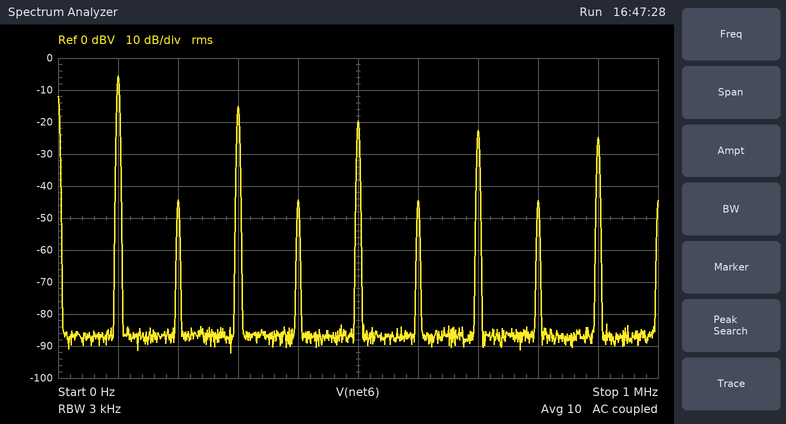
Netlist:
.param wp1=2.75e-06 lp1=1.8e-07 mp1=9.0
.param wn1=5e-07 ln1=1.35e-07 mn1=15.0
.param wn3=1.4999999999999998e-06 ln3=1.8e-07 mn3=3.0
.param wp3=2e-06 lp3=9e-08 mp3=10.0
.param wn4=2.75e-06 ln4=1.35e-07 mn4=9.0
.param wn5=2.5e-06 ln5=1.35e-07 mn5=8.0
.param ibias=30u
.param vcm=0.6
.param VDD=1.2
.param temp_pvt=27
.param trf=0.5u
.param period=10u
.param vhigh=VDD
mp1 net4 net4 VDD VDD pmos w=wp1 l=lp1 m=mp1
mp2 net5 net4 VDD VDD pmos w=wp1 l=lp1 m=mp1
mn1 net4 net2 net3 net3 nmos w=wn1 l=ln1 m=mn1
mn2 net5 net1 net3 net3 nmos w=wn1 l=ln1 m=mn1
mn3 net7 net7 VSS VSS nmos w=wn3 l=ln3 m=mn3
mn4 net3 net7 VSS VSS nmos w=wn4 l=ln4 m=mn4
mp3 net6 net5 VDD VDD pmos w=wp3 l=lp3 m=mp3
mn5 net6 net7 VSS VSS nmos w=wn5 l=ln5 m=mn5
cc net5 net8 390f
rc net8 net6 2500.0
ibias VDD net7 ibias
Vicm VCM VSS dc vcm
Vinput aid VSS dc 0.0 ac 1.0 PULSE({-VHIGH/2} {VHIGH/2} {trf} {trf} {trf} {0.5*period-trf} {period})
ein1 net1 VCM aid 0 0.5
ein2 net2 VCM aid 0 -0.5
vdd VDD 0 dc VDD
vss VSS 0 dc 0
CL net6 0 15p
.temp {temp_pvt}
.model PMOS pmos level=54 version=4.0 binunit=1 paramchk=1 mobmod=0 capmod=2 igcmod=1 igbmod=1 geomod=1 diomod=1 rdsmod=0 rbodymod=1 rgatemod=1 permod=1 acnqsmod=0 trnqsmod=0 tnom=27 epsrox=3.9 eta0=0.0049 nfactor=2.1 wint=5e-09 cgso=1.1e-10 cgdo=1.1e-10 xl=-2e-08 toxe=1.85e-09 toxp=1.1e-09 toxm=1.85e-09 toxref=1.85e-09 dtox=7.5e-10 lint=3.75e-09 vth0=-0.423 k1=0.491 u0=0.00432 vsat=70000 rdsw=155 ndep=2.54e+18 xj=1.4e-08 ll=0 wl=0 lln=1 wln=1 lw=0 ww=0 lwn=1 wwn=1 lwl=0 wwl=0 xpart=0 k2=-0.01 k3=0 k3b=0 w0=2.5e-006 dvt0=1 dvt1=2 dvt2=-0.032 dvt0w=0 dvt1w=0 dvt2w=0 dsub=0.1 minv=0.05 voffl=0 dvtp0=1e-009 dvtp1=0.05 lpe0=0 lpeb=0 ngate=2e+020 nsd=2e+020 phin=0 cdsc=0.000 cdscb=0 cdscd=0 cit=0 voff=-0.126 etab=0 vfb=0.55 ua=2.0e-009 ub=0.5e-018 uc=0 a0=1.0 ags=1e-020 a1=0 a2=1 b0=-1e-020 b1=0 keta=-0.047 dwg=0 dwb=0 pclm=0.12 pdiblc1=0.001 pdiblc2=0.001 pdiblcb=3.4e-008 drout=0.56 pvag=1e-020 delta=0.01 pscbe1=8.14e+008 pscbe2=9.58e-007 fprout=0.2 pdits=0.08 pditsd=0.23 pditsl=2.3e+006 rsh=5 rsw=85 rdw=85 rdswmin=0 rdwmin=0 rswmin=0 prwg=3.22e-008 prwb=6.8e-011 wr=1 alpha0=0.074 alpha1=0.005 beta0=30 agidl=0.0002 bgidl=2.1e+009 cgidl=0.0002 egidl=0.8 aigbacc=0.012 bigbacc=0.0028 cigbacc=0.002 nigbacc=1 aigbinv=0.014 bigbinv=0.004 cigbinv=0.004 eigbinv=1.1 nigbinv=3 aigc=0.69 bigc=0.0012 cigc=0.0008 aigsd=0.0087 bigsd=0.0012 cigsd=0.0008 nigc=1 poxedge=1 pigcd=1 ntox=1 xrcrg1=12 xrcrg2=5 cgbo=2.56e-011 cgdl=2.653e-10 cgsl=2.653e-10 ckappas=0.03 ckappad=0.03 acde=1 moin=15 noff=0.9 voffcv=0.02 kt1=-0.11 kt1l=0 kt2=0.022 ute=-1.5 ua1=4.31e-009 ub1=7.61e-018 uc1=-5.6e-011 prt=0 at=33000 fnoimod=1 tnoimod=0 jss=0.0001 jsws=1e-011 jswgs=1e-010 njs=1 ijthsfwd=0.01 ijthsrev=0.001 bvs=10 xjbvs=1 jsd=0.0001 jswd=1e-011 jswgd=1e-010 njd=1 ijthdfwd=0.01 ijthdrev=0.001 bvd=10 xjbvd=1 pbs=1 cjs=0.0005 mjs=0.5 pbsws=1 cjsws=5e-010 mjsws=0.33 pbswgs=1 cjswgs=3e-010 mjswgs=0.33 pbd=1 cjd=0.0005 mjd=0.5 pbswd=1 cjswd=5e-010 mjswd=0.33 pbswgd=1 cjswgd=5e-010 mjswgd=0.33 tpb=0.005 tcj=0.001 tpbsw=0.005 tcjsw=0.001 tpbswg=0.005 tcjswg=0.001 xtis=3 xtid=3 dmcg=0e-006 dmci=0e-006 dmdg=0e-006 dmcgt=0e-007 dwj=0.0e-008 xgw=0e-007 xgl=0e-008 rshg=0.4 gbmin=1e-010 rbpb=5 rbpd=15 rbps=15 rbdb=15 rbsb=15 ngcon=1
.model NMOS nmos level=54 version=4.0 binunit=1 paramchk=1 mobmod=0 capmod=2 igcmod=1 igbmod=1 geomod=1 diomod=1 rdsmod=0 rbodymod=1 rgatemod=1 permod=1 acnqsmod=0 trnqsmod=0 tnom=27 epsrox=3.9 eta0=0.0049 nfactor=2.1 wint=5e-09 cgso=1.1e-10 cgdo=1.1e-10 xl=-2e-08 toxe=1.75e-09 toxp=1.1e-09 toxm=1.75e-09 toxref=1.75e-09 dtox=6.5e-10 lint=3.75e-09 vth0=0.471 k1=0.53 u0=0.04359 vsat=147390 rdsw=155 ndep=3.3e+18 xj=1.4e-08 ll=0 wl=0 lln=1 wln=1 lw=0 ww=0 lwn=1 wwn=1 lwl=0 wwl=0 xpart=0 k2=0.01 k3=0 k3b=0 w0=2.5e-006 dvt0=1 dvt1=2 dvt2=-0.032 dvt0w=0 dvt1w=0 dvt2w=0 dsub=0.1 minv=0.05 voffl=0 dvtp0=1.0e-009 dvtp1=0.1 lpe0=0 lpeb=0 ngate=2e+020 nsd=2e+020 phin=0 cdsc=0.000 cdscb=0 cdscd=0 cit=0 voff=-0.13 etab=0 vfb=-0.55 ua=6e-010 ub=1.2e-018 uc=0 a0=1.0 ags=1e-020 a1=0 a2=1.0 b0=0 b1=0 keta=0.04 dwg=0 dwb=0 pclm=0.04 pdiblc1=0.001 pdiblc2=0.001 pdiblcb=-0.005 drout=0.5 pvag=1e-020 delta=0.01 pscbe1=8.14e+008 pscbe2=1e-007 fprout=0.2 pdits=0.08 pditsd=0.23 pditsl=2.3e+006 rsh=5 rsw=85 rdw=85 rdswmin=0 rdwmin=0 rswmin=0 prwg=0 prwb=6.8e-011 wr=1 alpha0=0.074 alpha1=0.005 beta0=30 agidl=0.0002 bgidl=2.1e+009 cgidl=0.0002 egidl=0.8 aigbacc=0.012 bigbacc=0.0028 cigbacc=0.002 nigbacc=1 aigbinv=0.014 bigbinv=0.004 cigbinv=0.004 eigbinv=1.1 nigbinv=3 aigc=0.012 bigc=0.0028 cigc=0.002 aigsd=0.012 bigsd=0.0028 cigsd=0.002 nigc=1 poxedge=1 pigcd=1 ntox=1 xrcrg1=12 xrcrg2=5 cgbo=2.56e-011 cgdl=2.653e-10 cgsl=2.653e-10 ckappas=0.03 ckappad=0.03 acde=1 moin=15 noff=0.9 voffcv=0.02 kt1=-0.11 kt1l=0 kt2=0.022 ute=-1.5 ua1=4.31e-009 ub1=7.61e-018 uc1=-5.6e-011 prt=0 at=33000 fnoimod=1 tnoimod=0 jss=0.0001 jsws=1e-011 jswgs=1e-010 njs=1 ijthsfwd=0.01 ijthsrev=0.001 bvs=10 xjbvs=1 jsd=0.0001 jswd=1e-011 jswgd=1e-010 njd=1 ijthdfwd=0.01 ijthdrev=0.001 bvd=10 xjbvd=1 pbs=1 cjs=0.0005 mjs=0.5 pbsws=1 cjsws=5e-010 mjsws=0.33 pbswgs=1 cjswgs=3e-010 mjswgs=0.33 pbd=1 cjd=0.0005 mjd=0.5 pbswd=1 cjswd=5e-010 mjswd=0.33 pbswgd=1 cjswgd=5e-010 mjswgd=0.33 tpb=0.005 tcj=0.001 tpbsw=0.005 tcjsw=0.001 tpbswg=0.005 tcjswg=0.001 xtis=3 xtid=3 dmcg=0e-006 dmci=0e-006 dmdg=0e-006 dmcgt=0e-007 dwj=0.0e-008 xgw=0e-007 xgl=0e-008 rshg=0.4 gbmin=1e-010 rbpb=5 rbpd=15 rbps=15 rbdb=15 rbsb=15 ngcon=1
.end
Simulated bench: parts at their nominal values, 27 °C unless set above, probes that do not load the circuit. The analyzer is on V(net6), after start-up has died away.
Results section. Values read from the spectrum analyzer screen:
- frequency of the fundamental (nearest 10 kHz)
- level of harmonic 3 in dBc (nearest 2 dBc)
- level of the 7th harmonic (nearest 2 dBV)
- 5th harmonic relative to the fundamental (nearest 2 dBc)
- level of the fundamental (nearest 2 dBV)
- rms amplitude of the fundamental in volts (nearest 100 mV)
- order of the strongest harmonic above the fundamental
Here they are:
100 kHz
-10 dBc
-22 dBV
-14 dBc
-6 dBV
500 mV
3
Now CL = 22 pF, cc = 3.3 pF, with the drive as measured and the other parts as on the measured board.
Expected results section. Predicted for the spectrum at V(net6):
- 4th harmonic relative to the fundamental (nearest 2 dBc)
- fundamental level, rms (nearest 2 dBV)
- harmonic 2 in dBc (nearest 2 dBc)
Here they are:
-34 dBc
-6 dBV
-34 dBc
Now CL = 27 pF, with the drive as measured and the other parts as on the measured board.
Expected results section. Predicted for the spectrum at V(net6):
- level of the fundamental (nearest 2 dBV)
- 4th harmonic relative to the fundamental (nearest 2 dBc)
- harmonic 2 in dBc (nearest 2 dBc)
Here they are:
-6 dBV
-34 dBc
-34 dBc
